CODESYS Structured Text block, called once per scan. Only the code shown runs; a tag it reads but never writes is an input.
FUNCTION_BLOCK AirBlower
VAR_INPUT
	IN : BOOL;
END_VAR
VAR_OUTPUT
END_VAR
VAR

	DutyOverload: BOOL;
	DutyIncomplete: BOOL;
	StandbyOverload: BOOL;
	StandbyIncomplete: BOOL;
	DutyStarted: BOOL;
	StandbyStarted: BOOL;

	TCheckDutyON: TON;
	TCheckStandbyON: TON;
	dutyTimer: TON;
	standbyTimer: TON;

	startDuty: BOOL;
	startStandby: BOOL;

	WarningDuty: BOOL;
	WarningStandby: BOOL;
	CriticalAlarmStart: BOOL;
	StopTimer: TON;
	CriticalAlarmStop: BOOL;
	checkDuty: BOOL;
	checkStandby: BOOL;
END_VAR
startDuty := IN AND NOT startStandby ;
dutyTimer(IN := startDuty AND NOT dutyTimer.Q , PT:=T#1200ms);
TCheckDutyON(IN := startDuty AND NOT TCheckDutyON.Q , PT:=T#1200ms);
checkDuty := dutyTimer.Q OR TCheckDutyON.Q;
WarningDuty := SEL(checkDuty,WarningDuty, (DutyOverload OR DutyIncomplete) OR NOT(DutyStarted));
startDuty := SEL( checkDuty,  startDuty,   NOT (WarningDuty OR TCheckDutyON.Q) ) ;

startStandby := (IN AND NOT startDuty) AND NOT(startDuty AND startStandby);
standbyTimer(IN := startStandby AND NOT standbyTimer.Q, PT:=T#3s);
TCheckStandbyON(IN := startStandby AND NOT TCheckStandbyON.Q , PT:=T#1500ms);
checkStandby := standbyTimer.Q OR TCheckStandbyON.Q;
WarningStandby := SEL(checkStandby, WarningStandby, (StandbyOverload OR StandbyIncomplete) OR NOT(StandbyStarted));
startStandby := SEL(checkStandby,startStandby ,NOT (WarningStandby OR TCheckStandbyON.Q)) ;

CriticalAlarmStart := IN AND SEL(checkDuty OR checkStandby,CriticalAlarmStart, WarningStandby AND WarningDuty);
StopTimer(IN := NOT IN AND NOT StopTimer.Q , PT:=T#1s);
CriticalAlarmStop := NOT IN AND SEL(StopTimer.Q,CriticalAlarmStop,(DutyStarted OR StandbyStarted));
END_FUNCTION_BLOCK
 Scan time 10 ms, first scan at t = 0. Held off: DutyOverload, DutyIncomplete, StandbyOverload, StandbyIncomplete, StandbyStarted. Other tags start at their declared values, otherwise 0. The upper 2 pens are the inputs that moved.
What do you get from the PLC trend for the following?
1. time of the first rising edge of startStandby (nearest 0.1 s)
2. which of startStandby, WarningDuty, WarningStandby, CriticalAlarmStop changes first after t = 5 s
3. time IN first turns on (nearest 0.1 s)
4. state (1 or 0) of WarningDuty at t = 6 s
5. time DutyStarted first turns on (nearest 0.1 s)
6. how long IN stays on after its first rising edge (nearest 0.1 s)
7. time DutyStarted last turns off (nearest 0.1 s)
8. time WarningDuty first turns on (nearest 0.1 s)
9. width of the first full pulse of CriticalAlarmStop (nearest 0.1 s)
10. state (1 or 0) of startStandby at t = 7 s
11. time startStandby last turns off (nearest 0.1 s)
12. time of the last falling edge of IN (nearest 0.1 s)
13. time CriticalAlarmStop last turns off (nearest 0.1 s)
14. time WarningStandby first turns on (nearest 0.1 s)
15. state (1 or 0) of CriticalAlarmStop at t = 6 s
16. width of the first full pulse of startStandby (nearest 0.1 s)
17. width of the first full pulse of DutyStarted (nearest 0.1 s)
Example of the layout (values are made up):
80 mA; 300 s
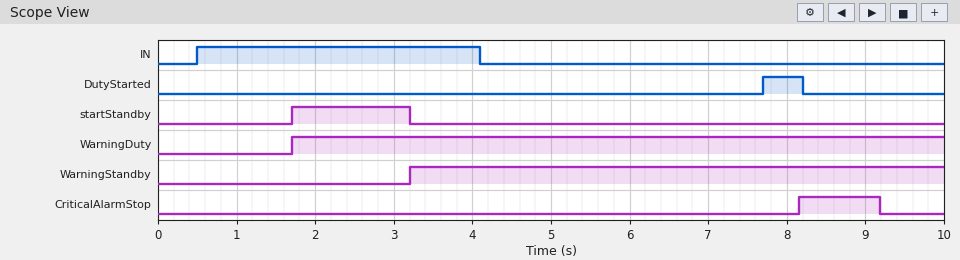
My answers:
1.7 s; CriticalAlarmStop; 0.5 s; 1; 7.7 s; 3.6 s; 8.2 s; 1.7 s; 1.0 s; 0; 3.2 s; 4.1 s; 9.2 s; 3.2 s; 0; 1.5 s; 0.5 s
